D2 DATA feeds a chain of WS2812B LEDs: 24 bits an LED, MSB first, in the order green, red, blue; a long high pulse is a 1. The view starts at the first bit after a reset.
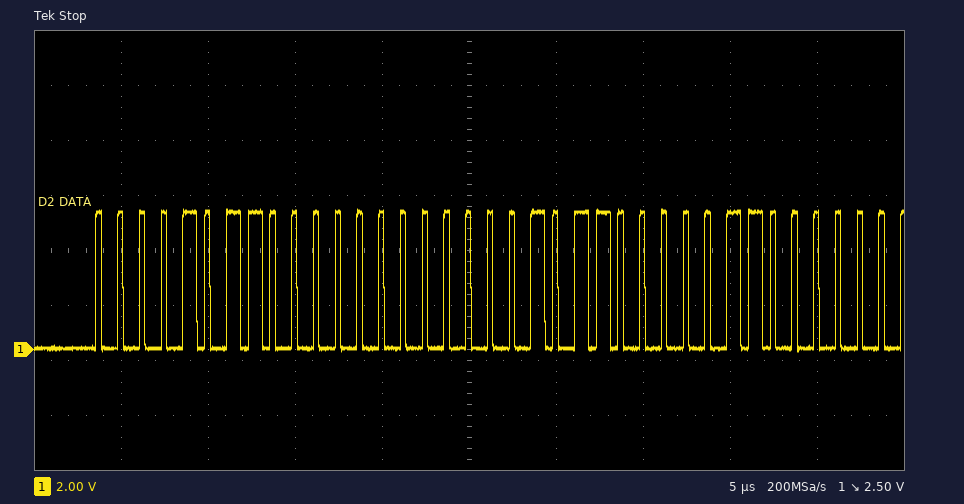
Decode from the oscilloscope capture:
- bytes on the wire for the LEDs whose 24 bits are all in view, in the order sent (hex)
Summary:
0B 00 0B
